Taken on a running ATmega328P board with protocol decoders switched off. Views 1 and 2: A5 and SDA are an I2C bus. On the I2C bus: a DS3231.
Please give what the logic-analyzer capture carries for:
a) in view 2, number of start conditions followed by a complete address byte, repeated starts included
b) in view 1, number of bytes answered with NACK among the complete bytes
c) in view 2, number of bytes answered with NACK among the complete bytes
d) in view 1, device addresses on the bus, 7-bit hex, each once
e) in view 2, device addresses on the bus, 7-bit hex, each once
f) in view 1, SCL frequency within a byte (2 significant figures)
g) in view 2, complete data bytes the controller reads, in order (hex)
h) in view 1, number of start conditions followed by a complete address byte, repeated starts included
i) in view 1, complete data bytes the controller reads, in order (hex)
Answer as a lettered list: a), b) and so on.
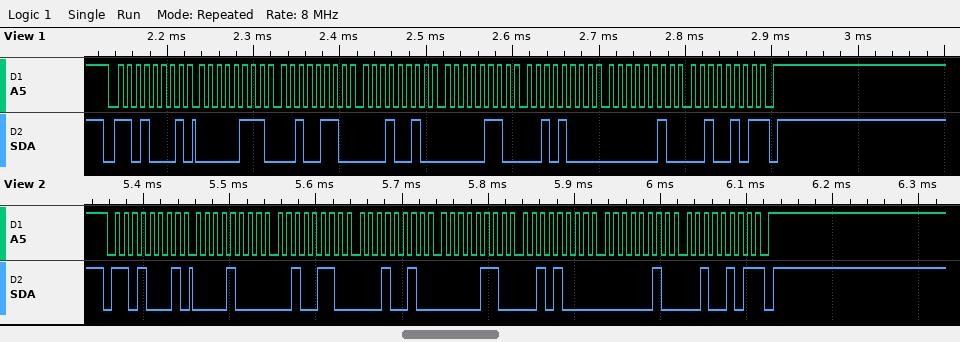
a) 1
b) 1
c) 1
d) 0x68
e) 0x68
f) 100 kHz
g) 08 26 12 06 28 02 25
h) 1
i) 07 26 12 06 28 02 25
